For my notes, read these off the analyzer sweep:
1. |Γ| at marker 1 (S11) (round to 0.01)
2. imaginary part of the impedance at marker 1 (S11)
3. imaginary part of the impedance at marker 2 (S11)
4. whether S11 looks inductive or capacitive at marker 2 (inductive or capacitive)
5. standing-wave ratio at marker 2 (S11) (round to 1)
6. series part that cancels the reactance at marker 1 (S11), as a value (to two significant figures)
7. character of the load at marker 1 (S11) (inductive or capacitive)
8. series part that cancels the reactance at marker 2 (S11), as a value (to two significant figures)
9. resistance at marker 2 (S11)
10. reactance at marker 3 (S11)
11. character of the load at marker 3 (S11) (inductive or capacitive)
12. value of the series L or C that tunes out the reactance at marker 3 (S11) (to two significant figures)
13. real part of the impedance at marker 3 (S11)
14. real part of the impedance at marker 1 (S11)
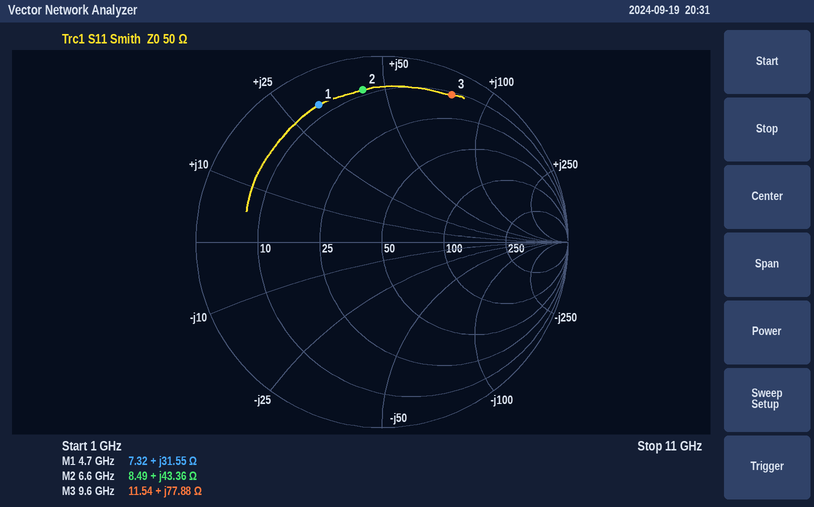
0.81
+31.55 Ω
+43.36 Ω
inductive
10
1.1 pF
inductive
560 fF
8.49 Ω
+77.88 Ω
inductive
210 fF
11.54 Ω
7.32 Ω
